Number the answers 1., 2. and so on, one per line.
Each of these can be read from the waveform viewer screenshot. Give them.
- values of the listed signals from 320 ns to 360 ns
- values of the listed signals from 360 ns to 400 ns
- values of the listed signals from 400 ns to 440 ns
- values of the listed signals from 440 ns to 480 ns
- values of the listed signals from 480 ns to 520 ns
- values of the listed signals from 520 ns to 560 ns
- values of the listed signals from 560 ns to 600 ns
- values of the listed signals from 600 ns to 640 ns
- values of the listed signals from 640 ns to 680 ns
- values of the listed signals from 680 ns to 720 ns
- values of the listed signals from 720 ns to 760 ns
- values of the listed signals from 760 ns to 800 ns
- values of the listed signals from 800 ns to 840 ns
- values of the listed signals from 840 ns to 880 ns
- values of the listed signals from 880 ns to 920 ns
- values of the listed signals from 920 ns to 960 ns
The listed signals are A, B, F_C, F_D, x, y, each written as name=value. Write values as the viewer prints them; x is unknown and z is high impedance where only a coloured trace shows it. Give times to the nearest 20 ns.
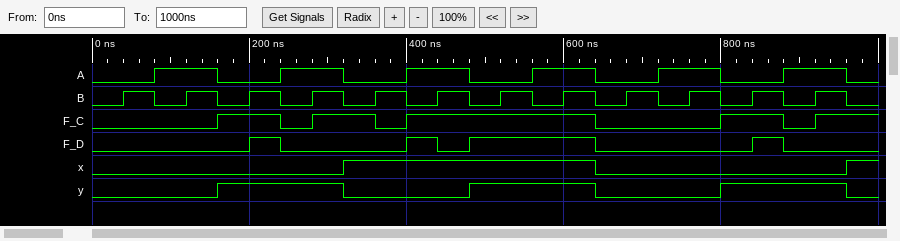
1. A=0, B=0, F_C=1, F_D=0, x=1, y=0
2. A=0, B=1, F_C=0, F_D=0, x=1, y=0
3. A=1, B=0, F_C=1, F_D=1, x=1, y=0
4. A=1, B=1, F_C=1, F_D=0, x=1, y=0
5. A=0, B=0, F_C=1, F_D=1, x=1, y=1
6. A=0, B=1, F_C=1, F_D=1, x=1, y=1
7. A=1, B=0, F_C=1, F_D=1, x=1, y=1
8. A=1, B=1, F_C=1, F_D=1, x=1, y=1
9. A=0, B=0, F_C=0, F_D=0, x=0, y=0
10. A=0, B=1, F_C=0, F_D=0, x=0, y=0
11. A=1, B=0, F_C=0, F_D=0, x=0, y=0
12. A=1, B=1, F_C=0, F_D=0, x=0, y=0
13. A=0, B=0, F_C=1, F_D=0, x=0, y=1
14. A=0, B=1, F_C=1, F_D=1, x=0, y=1
15. A=1, B=0, F_C=0, F_D=0, x=0, y=1
16. A=1, B=1, F_C=1, F_D=0, x=0, y=1
